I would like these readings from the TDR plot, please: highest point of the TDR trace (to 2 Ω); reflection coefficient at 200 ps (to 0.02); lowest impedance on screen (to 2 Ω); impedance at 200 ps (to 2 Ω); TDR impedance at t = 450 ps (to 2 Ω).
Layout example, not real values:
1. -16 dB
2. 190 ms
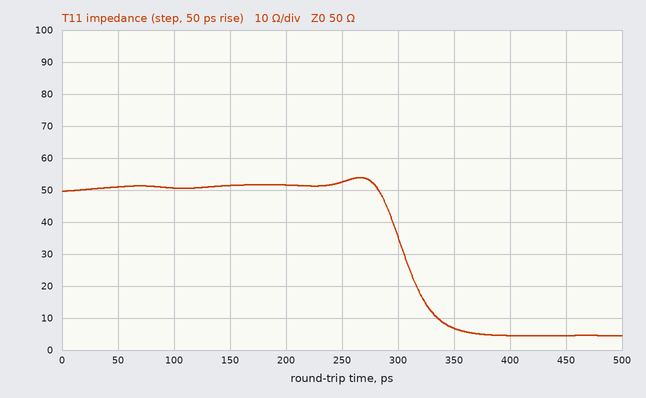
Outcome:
1. 54 Ω
2. +0.02
3. 4 Ω
4. 52 Ω
5. 4 Ω
